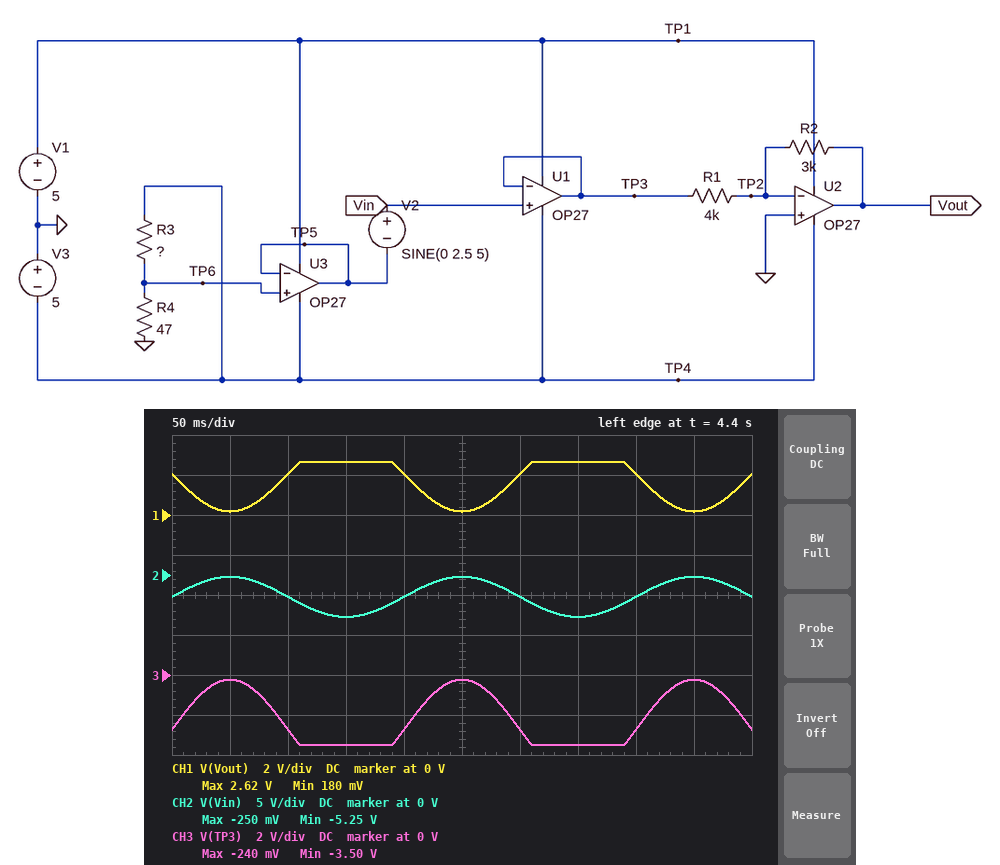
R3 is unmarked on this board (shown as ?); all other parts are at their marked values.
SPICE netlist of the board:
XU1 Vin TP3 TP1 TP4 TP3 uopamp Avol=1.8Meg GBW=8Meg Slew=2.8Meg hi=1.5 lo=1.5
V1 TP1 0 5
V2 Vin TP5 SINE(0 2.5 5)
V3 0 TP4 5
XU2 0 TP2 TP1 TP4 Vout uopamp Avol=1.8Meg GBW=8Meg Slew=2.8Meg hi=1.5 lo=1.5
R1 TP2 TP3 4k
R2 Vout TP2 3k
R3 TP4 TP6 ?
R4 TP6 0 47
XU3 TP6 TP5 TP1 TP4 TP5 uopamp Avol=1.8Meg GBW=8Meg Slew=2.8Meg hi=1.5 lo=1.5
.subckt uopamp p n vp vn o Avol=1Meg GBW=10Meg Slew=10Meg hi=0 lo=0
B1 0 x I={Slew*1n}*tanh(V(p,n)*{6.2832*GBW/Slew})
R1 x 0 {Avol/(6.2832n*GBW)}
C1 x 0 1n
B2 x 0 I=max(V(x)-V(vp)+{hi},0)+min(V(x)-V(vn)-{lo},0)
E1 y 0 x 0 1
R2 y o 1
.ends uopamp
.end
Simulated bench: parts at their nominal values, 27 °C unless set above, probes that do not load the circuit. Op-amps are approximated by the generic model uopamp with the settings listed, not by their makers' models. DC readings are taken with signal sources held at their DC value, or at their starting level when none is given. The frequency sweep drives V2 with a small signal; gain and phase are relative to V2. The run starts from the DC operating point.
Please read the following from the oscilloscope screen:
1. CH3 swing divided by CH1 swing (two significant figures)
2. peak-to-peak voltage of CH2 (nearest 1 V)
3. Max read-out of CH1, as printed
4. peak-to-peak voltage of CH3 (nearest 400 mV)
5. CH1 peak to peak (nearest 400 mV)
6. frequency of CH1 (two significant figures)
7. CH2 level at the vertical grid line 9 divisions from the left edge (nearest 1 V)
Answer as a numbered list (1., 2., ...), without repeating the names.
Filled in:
1. 1.3
2. 5 V
3. 2.62 V
4. 3.2 V
5. 2.4 V
6. 5.0 Hz
7. 0 V
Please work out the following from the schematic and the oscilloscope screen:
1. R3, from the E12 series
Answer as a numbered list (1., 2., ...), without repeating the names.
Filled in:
1. 39 Ω
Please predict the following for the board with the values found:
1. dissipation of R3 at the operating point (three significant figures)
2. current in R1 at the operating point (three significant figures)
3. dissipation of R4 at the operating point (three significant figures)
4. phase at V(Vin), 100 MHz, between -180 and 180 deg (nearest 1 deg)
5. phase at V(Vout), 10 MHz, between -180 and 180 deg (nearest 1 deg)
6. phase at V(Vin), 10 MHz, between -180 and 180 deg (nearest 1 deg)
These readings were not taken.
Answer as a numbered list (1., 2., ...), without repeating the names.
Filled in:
1. 132 mW
2. 683 µA
3. 159 mW
4. 0 deg
5. 63 deg
6. 0 deg
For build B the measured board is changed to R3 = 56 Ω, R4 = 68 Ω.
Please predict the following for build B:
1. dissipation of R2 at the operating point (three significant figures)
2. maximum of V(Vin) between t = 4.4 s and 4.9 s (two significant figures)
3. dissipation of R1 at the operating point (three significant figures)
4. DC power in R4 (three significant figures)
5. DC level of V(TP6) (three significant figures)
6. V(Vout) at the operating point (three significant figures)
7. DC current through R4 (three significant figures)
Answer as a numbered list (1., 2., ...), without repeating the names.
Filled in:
1. 1.41 mW
2. -240 mV
3. 1.88 mW
4. 111 mW
5. -2.74 V
6. 2.06 V
7. 40.3 mA
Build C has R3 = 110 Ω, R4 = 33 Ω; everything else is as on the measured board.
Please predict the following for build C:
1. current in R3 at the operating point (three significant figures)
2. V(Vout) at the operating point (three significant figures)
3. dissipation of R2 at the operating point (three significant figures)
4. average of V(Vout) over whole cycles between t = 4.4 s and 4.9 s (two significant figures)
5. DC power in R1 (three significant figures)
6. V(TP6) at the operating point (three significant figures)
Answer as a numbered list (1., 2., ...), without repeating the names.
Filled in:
1. 35.0 mA
2. 865 mV
3. 250 µW
4. 860 mV
5. 333 µW
6. -1.15 V
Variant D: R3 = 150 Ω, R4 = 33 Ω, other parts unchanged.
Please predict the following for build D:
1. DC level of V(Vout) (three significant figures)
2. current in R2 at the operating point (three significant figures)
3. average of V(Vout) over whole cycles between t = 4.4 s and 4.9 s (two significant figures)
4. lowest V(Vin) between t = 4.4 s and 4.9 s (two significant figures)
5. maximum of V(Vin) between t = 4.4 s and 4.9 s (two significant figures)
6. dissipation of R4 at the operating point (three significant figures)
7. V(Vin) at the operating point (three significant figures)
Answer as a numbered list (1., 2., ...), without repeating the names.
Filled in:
1. 676 mV
2. 225 µA
3. 680 mV
4. -3.4 V
5. 1.6 V
6. 24.6 mW
7. -902 mV
